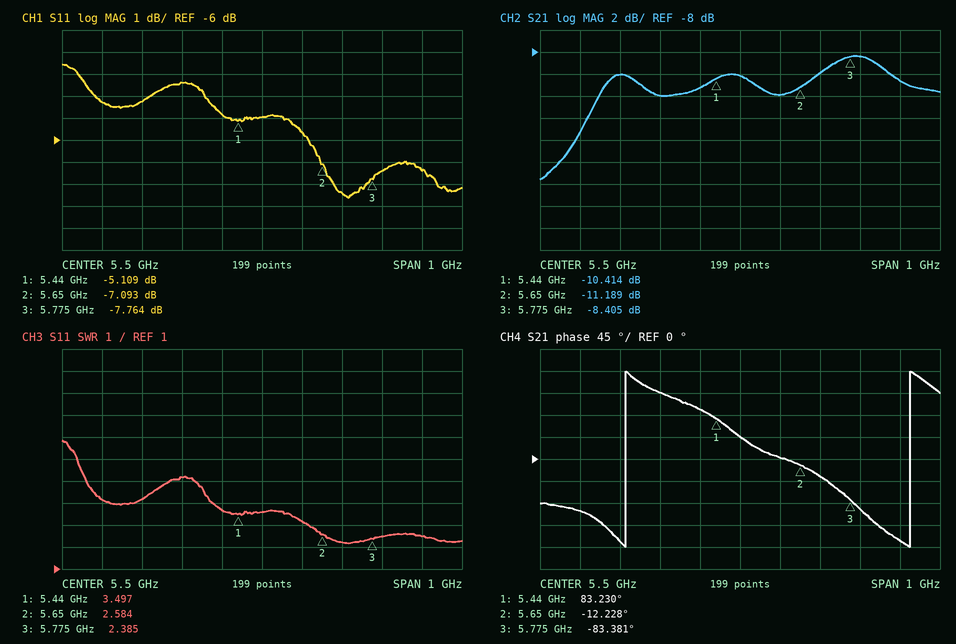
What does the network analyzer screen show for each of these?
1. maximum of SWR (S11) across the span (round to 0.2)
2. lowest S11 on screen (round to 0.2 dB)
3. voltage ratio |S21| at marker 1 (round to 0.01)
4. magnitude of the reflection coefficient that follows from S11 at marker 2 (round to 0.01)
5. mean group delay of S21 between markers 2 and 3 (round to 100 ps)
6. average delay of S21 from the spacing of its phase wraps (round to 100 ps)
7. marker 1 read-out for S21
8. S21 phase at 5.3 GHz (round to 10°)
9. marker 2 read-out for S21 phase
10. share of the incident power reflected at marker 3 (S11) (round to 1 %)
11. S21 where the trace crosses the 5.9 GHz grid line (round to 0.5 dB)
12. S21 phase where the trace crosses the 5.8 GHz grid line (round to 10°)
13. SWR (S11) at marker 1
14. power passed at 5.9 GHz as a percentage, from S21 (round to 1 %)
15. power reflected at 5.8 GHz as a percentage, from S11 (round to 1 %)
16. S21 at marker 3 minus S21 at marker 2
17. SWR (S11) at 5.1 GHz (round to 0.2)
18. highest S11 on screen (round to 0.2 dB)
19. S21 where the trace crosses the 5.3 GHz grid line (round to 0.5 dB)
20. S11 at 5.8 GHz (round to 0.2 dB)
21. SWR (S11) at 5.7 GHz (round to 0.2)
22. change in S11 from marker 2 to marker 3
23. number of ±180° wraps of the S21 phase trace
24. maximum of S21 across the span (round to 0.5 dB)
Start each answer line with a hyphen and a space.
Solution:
- 6.8
- -8.6 dB
- 0.30
- 0.44
- 1.6 ns
- 1.4 ns
- -10.414 dB
- 140°
- -12.228°
- 17 %
- -10.5 dB
- -100°
- 3.497
- 9 %
- 18 %
- 2.784 dB
- 4.2
- -2.6 dB
- -12.0 dB
- -7.4 dB
- 2.2
- -0.671 dB
- 2
- -8.5 dB
